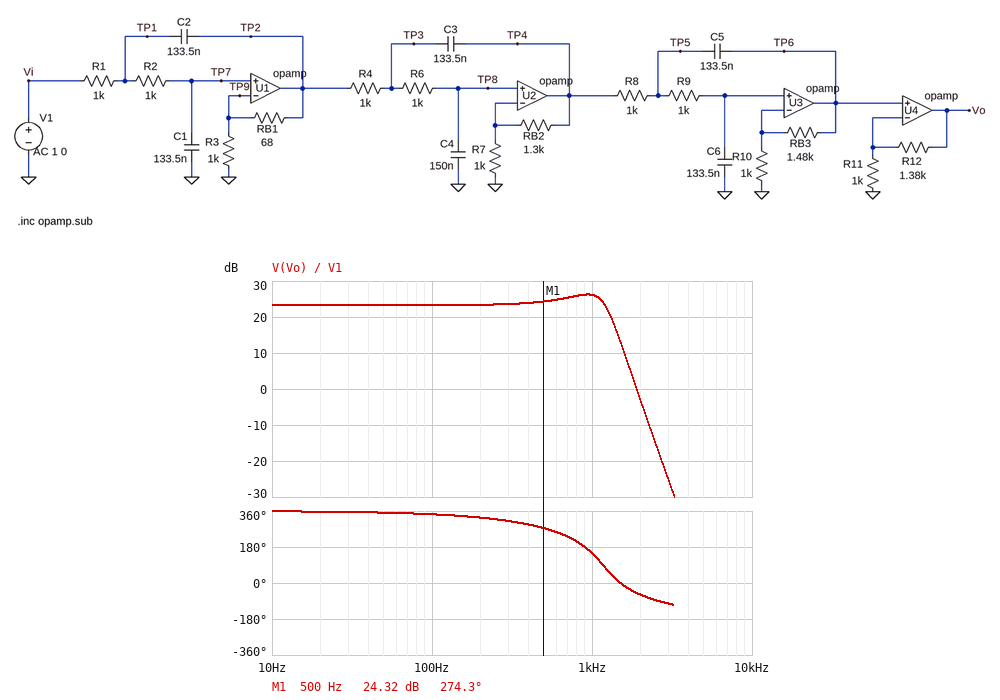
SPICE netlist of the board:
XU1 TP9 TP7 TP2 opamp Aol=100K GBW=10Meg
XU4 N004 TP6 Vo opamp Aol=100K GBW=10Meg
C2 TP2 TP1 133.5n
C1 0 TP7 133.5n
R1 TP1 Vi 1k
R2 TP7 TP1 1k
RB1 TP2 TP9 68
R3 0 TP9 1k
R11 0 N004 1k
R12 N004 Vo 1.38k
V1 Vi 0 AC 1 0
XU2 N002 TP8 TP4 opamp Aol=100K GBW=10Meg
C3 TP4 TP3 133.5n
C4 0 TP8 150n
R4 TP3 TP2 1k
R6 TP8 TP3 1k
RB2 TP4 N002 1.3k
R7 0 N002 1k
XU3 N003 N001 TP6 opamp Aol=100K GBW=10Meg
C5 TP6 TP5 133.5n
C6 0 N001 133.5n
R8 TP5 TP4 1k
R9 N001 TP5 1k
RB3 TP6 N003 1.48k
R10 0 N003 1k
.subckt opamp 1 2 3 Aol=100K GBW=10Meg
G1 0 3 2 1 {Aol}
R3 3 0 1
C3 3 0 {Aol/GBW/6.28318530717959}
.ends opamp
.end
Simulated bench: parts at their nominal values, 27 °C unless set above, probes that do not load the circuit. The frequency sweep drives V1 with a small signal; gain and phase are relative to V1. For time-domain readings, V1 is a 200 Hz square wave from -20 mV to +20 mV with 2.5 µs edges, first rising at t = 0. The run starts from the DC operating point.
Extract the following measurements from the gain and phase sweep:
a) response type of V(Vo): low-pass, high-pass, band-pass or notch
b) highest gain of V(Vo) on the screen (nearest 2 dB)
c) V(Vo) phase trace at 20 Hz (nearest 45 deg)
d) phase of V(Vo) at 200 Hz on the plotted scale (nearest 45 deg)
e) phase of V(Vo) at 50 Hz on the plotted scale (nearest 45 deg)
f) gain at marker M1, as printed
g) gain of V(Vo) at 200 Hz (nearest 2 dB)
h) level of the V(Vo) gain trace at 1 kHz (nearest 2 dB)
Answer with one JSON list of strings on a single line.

["low-pass", "26 dB", "360 deg", "315 deg", "360 deg", "24.32 dB", "24 dB", "26 dB"]
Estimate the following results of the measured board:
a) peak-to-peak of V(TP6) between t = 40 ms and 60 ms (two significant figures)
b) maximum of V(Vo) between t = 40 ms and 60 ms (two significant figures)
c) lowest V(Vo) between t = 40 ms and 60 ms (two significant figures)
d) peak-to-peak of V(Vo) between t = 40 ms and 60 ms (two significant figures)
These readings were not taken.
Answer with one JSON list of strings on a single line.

["390 mV", "460 mV", "-460 mV", "930 mV"]
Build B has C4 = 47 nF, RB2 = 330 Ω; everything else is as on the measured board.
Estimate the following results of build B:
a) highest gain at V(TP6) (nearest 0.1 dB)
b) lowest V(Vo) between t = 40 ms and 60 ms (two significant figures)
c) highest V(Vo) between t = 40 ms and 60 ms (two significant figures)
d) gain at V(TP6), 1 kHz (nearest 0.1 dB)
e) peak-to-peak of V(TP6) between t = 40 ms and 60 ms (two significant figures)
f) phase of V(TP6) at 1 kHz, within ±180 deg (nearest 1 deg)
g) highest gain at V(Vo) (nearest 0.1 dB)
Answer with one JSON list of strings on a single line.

["14.1 dB", "-260 mV", "260 mV", "13.9 dB", "220 mV", "-158 deg", "21.6 dB"]
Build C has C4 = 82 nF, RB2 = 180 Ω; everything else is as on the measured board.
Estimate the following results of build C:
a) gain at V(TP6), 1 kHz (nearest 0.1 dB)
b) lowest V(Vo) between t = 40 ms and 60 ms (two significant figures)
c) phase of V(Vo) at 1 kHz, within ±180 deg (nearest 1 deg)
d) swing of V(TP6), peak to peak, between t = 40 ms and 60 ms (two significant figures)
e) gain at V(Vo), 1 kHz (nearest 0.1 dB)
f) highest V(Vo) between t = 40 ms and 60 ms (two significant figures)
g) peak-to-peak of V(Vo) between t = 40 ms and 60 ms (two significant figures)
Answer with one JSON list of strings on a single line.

["10.7 dB", "-200 mV", "167 deg", "170 mV", "18.3 dB", "200 mV", "400 mV"]
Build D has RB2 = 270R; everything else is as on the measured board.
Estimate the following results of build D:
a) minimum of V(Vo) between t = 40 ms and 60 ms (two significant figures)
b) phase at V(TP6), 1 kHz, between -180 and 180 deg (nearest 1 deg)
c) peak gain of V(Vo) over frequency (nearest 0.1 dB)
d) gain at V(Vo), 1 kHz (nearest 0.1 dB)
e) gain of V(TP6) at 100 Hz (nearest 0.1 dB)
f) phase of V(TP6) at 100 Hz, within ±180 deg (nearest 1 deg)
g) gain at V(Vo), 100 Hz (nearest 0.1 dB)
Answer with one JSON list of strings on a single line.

["-170 mV", "142 deg", "18.1 dB", "14.8 dB", "10.5 dB", "-21 deg", "18.0 dB"]
